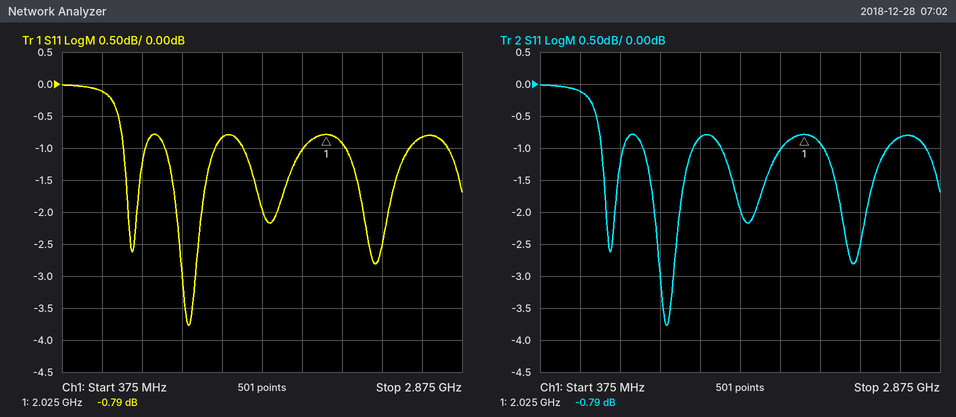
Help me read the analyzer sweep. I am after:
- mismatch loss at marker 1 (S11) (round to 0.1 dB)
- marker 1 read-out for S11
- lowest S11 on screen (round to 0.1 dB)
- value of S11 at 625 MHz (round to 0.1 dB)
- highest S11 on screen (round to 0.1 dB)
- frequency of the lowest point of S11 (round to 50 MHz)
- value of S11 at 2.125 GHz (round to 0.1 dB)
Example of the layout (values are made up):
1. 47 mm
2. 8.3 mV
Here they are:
1. 7.8 dB
2. -0.79 dB
3. -3.8 dB
4. -0.1 dB
5. 0.0 dB
6. 1.15 GHz
7. -0.9 dB
